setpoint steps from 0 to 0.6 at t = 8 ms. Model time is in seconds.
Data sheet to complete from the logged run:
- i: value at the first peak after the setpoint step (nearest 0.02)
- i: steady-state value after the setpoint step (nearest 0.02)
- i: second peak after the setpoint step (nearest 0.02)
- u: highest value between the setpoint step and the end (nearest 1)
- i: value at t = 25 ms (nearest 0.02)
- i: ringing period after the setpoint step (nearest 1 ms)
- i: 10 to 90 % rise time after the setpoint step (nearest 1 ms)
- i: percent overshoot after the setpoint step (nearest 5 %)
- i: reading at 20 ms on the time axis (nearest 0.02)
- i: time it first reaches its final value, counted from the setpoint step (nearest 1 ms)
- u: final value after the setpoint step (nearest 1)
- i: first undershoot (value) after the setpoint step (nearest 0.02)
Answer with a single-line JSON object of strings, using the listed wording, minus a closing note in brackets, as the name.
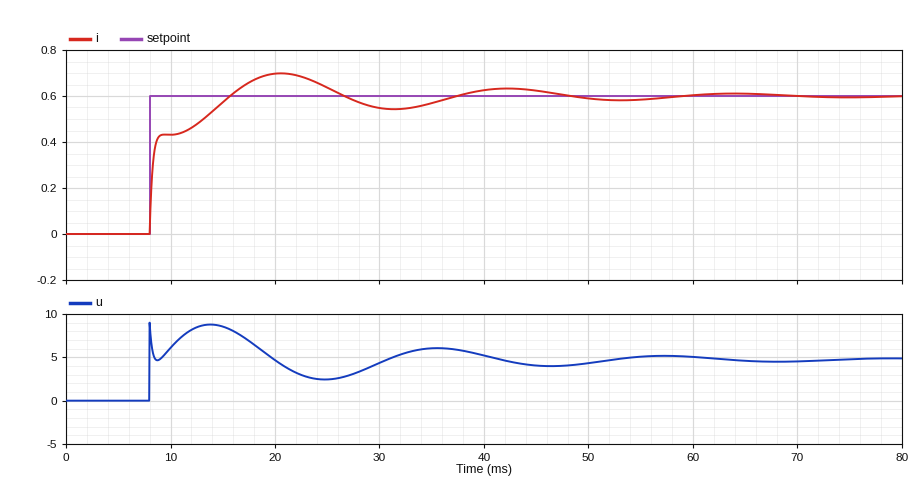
{"i: value at the first peak after the setpoint step": "0.70", "i: steady-state value after the setpoint step": "0.60", "i: second peak after the setpoint step": "0.64", "u: highest value between the setpoint step and the end": "9", "i: value at t = 25 ms": "0.64", "i: ringing period after the setpoint step": "22 ms", "i: 10 to 90 % rise time after the setpoint step": "6 ms", "i: percent overshoot after the setpoint step": "15 %", "i: reading at 20 ms on the time axis": "0.70", "i: time it first reaches its final value, counted from the setpoint step": "8 ms", "u: final value after the setpoint step": "5", "i: first undershoot (value) after the setpoint step": "0.54"}
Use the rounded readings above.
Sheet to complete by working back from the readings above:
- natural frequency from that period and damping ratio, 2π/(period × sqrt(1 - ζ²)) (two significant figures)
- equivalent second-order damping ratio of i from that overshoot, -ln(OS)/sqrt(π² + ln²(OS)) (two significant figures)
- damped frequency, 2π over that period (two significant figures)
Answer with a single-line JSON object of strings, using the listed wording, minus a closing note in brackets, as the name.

{"natural frequency from that period and damping ratio, 2π/(period × sqrt(1 - ζ²))": "0.33 rad/ms", "equivalent second-order damping ratio of i from that overshoot, -ln(OS)/sqrt(π² + ln²(OS))": "0.52", "damped frequency, 2π over that period": "0.29 rad/ms"}
